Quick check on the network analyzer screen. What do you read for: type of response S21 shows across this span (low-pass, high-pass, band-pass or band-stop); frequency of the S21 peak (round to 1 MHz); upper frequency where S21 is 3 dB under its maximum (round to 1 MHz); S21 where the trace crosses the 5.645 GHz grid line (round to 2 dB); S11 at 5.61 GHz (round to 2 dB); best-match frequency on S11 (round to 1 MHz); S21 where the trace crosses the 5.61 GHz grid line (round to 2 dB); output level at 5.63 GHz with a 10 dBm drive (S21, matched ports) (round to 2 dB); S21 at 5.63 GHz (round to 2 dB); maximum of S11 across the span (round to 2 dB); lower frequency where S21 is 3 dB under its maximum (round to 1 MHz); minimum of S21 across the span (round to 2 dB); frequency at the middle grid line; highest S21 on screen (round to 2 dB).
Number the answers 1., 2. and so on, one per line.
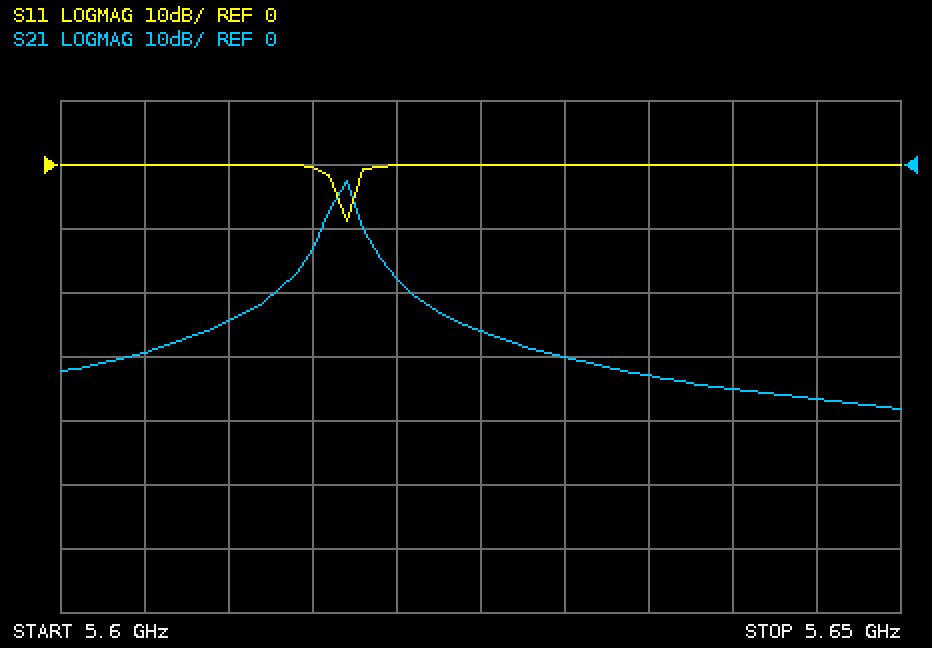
1. band-pass
2. 5.617 GHz
3. 5.617 GHz
4. -36 dB
5. 0 dB
6. 5.617 GHz
7. -24 dB
8. -20 dBm
9. -30 dB
10. 0 dB
11. 5.616 GHz
12. -38 dB
13. 5.625 GHz
14. -2 dB
